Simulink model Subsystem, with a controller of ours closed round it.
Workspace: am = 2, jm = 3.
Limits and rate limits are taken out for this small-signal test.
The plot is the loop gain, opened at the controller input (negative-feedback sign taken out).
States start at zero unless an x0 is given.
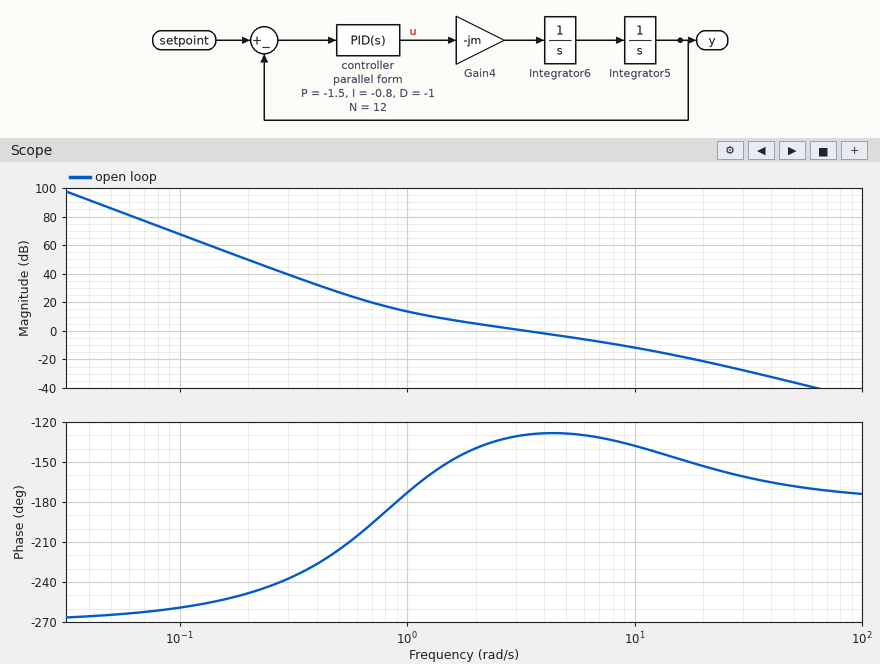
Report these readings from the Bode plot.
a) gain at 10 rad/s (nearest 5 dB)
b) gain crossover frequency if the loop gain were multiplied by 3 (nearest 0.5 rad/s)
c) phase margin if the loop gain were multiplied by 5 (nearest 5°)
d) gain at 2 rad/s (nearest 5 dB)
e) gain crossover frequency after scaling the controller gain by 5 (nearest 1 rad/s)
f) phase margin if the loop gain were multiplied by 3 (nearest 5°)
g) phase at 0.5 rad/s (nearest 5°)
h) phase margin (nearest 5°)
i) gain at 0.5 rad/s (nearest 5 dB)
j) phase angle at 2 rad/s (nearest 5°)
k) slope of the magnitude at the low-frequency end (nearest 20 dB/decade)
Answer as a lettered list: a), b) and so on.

a) -10 dB
b) 8.5 rad/s
c) 40°
d) 5 dB
e) 12 rad/s
f) 45°
g) -215°
h) 50°
i) 25 dB
j) -140°
k) -60 dB/decade
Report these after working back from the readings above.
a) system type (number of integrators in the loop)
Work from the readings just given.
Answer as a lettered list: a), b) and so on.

a) 3
